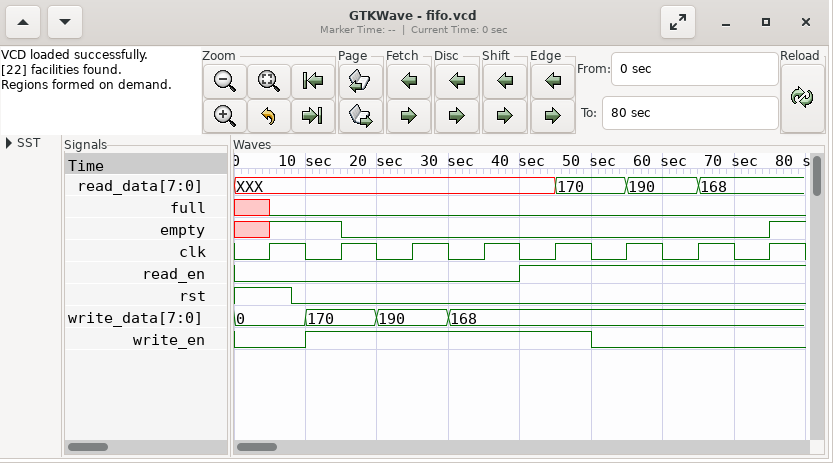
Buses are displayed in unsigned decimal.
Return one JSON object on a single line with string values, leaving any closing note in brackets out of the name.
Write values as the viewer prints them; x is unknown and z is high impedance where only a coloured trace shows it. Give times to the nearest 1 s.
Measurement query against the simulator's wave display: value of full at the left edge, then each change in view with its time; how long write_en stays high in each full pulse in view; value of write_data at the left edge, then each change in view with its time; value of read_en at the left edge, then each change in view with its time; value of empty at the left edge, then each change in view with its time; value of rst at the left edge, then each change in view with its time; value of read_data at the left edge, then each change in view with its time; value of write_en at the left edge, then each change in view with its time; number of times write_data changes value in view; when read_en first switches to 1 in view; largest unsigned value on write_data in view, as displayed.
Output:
{"value of full at the left edge, then each change in view with its time": "x, 0 at 5 s", "how long write_en stays high in each full pulse in view": "40 s", "value of write_data at the left edge, then each change in view with its time": "0, 170 at 10 s, 190 at 20 s, 168 at 30 s", "value of read_en at the left edge, then each change in view with its time": "0, 1 at 40 s", "value of empty at the left edge, then each change in view with its time": "x, 1 at 5 s, 0 at 15 s, 1 at 75 s", "value of rst at the left edge, then each change in view with its time": "1, 0 at 8 s", "value of read_data at the left edge, then each change in view with its time": "XXX, 170 at 45 s, 190 at 55 s, 168 at 65 s", "value of write_en at the left edge, then each change in view with its time": "0, 1 at 10 s, 0 at 50 s", "number of times write_data changes value in view": "3", "when read_en first switches to 1 in view": "40 s", "largest unsigned value on write_data in view, as displayed": "190"}
